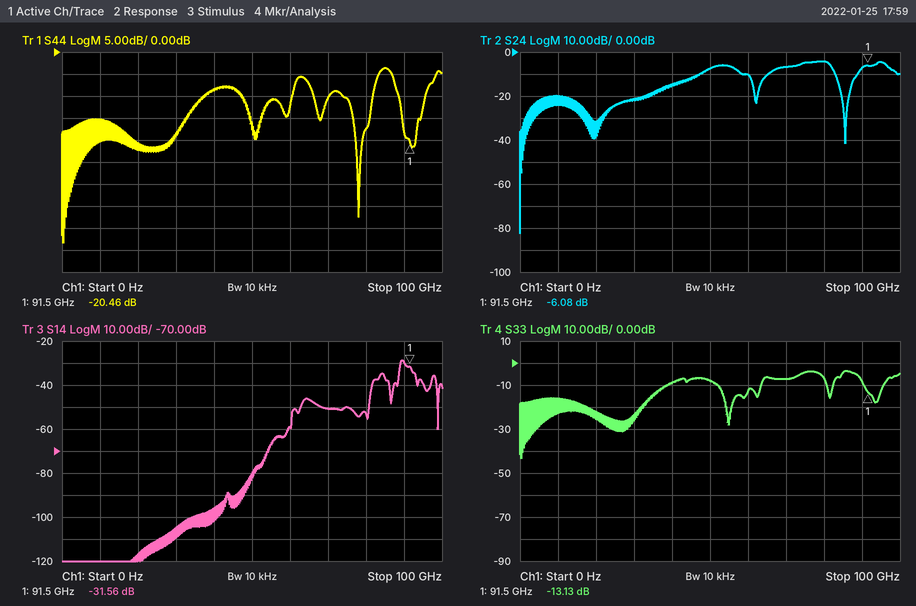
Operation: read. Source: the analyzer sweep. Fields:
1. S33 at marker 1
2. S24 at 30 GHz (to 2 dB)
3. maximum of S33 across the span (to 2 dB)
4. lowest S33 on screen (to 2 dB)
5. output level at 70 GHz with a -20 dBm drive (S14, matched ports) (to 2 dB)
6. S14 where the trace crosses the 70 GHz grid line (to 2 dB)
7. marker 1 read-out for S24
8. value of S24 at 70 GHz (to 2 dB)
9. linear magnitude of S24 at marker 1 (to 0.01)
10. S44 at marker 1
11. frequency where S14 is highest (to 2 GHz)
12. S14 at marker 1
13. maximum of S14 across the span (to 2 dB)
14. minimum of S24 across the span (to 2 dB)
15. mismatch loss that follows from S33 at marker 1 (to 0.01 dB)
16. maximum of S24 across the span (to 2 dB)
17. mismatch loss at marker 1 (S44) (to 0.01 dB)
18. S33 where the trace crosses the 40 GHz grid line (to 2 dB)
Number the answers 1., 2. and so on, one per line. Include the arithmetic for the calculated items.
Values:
1. -13.13 dB
2. -22 dB
3. -4 dB
4. -44 dB
5. -20 dBm + (-50 dB) = -70 dBm
6. -50 dB
7. -6.08 dB
8. -6 dB
9. 10^(-6.08/20) ≈ 0.50
10. -20.46 dB
11. 90 GHz
12. -31.56 dB
13. -28 dB
14. -82 dB
15. −10 log10(1 − 10^(-13.13/10)) ≈ 0.22 dB
16. -4 dB
17. −10 log10(1 − 10^(-20.46/10)) ≈ 0.04 dB
18. -8 dB
